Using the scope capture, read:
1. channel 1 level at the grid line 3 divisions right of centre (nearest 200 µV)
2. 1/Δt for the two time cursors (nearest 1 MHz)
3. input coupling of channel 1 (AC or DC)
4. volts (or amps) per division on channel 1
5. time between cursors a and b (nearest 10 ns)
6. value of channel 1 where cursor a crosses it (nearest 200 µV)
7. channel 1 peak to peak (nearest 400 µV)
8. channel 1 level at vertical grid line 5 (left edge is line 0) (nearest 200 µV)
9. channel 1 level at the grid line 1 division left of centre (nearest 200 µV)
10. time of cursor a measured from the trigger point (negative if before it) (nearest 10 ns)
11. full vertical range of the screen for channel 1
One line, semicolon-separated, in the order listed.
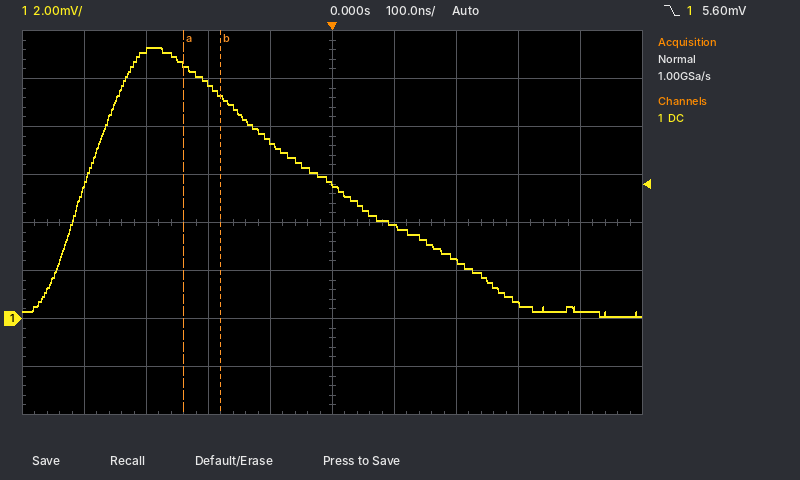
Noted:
600 µV; 17 MHz; DC; 2 mV; 60 ns; 10.6 mV; 11.2 mV; 5.6 mV; 7.4 mV; -240 ns; 16 mV
